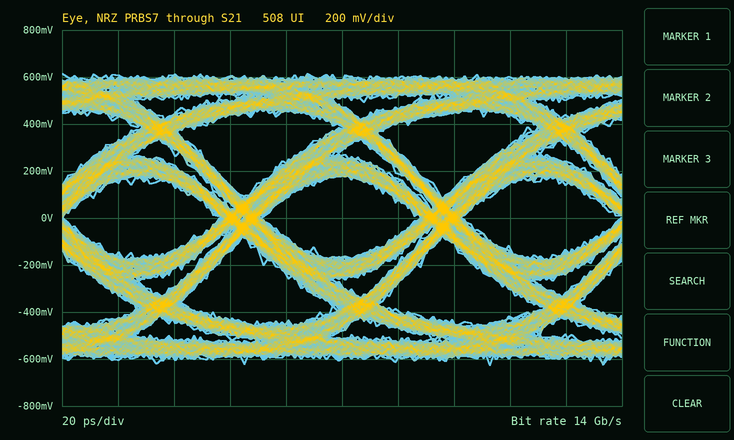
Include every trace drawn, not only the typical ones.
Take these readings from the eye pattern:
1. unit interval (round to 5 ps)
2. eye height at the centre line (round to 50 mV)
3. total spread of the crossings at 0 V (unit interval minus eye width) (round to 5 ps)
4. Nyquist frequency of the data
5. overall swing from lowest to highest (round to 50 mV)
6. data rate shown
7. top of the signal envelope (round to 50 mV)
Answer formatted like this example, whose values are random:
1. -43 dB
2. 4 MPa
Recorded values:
1. 70 ps
2. 350 mV
3. 15 ps
4. 7 GHz
5. 1.25 V
6. 14 Gb/s
7. 600 mV
